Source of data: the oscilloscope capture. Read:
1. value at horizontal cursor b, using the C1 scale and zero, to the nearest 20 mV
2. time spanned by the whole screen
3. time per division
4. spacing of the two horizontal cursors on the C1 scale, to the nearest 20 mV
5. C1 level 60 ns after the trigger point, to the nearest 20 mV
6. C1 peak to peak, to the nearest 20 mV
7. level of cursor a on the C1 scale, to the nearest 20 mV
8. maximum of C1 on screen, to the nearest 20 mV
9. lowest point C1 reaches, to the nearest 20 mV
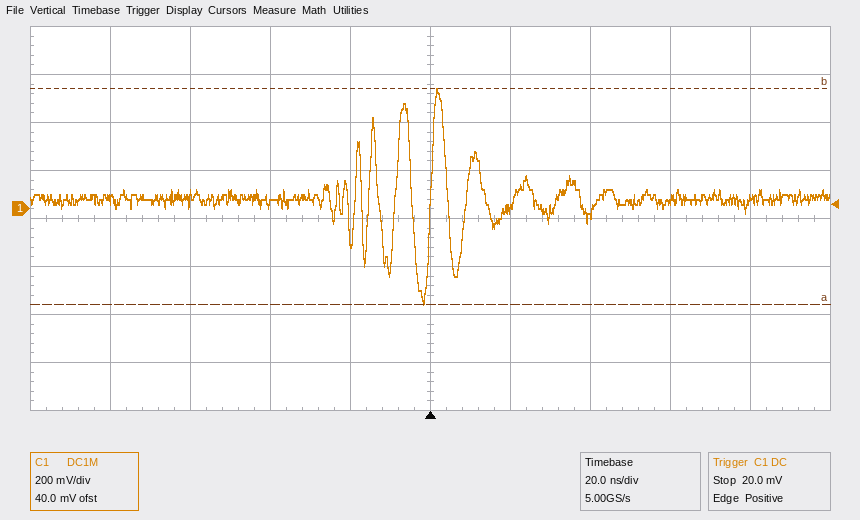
500 mV
200 ns
20 ns
900 mV
40 mV
900 mV
-400 mV
500 mV
-400 mV
